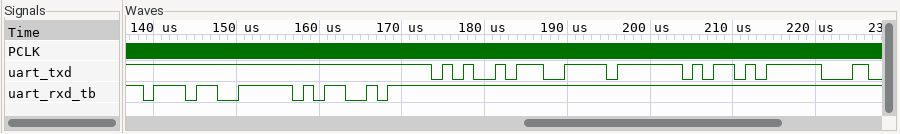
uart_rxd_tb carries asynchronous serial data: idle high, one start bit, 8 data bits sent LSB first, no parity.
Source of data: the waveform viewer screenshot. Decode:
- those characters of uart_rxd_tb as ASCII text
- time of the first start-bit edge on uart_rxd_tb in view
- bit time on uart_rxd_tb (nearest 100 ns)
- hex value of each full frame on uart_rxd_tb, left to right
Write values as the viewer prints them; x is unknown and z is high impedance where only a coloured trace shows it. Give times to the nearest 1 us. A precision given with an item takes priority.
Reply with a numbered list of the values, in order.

1. "7M"
2. 139 us
3. 1300 ns
4. 37, 4D
